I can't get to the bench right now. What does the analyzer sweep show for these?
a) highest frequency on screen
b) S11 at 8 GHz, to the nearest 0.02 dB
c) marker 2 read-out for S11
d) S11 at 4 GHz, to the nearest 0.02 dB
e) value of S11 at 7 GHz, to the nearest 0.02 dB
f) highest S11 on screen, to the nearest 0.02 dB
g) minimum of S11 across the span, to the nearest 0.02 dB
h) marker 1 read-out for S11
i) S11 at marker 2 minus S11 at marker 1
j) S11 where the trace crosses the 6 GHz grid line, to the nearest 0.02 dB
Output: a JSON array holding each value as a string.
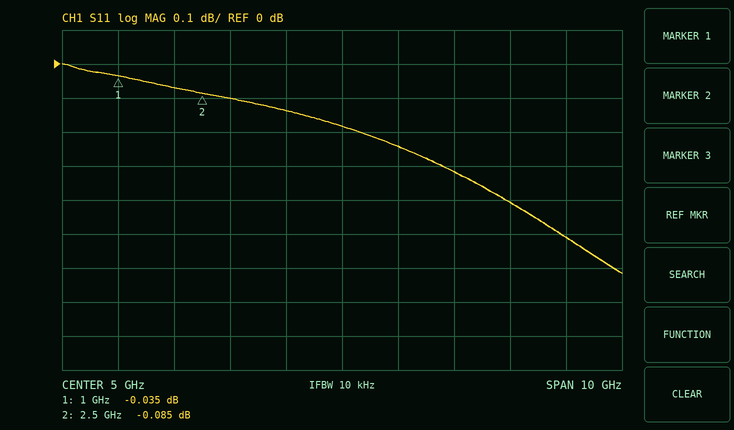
["10 GHz", "-0.40 dB", "-0.085 dB", "-0.14 dB", "-0.32 dB", "0.00 dB", "-0.62 dB", "-0.035 dB", "-0.050 dB", "-0.24 dB"]
